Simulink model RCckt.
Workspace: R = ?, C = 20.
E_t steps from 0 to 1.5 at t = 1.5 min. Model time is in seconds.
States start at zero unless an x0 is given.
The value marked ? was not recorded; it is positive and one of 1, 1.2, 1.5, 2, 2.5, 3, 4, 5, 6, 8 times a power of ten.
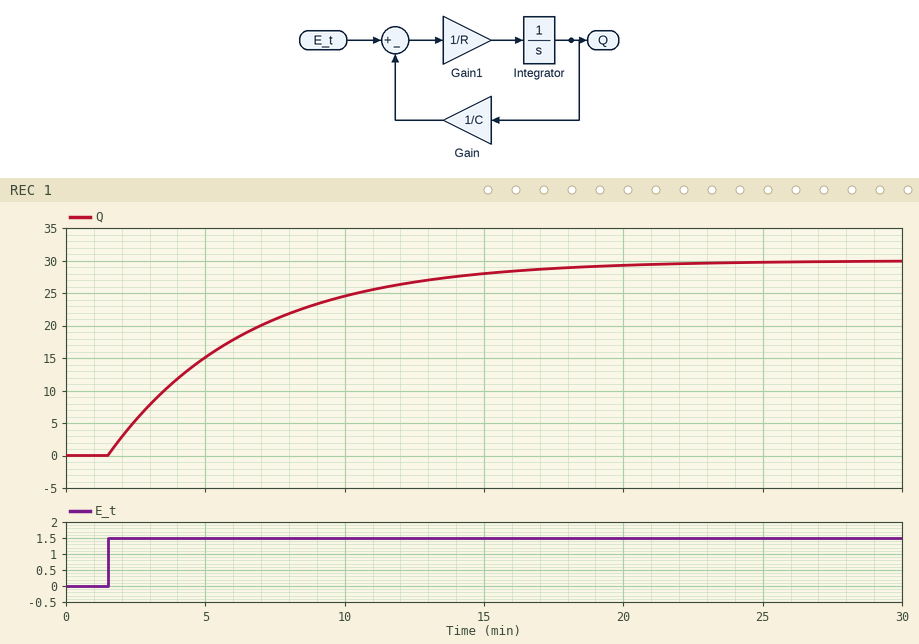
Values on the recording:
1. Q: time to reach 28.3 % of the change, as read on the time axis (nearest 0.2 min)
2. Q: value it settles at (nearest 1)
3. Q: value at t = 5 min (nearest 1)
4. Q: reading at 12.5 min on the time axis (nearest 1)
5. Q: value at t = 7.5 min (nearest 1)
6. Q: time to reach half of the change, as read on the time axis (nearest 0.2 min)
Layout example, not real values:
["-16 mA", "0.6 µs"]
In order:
["3.2 min", "30", "15", "27", "21", "5.0 min"]
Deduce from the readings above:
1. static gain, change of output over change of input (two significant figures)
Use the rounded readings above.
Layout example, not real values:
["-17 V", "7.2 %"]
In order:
["20"]
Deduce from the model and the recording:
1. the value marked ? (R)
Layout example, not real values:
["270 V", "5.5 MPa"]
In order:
["15"]
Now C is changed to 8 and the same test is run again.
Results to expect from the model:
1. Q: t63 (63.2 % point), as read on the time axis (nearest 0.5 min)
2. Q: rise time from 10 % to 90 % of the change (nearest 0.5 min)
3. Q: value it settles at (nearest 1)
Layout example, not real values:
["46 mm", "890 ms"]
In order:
["3.5 min", "4.5 min", "12"]
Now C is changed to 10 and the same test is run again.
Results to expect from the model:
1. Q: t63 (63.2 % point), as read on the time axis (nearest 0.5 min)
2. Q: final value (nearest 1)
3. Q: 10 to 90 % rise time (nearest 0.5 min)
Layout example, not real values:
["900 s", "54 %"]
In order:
["4.0 min", "15", "5.5 min"]
